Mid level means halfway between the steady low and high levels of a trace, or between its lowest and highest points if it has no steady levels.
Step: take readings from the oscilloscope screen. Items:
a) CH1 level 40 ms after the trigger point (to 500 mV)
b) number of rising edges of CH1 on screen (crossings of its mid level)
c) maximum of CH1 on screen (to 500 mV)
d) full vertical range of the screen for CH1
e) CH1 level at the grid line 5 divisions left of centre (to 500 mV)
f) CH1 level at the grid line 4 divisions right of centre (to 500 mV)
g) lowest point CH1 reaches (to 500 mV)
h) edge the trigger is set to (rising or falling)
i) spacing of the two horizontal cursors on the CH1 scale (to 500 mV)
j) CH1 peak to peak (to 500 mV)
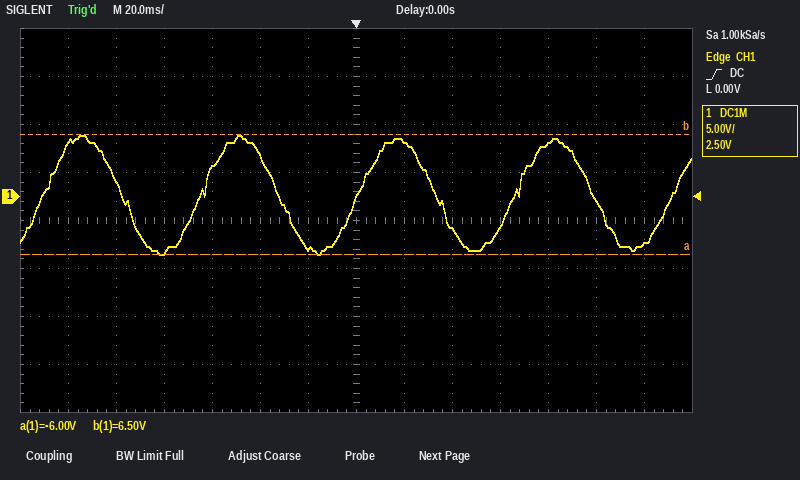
-3.5 V
5
6.5 V
40 V
1.5 V
5.5 V
-6.0 V
rising
12.5 V
12.5 V
